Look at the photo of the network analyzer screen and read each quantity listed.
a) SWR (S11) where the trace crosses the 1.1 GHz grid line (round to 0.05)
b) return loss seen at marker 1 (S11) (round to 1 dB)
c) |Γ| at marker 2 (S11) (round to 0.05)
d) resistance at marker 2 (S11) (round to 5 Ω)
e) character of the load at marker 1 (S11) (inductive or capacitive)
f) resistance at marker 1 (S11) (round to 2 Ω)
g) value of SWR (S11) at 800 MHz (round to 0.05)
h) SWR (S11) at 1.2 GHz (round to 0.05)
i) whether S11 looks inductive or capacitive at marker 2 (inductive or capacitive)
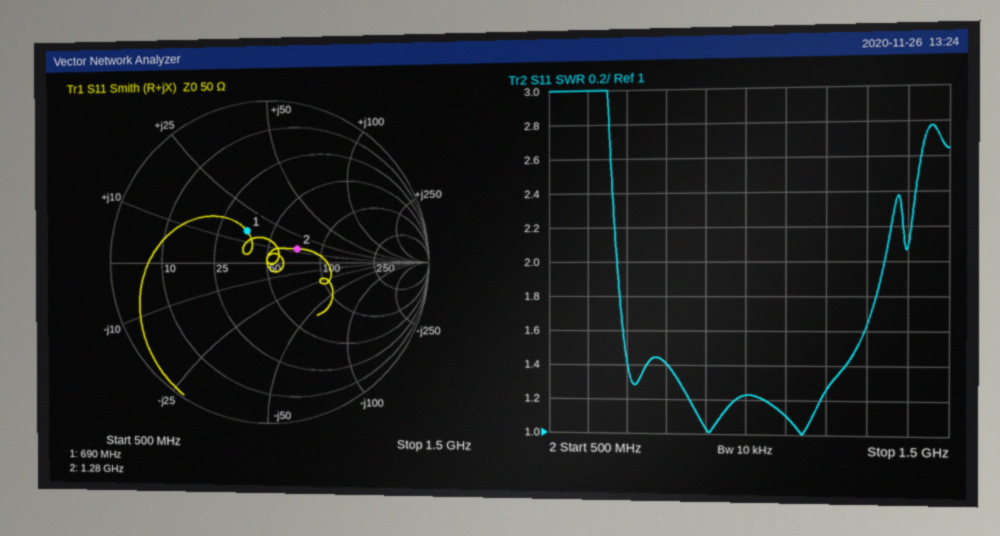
1.10
13 dB
0.20
70 Ω
inductive
36 Ω
1.40
1.25
inductive
